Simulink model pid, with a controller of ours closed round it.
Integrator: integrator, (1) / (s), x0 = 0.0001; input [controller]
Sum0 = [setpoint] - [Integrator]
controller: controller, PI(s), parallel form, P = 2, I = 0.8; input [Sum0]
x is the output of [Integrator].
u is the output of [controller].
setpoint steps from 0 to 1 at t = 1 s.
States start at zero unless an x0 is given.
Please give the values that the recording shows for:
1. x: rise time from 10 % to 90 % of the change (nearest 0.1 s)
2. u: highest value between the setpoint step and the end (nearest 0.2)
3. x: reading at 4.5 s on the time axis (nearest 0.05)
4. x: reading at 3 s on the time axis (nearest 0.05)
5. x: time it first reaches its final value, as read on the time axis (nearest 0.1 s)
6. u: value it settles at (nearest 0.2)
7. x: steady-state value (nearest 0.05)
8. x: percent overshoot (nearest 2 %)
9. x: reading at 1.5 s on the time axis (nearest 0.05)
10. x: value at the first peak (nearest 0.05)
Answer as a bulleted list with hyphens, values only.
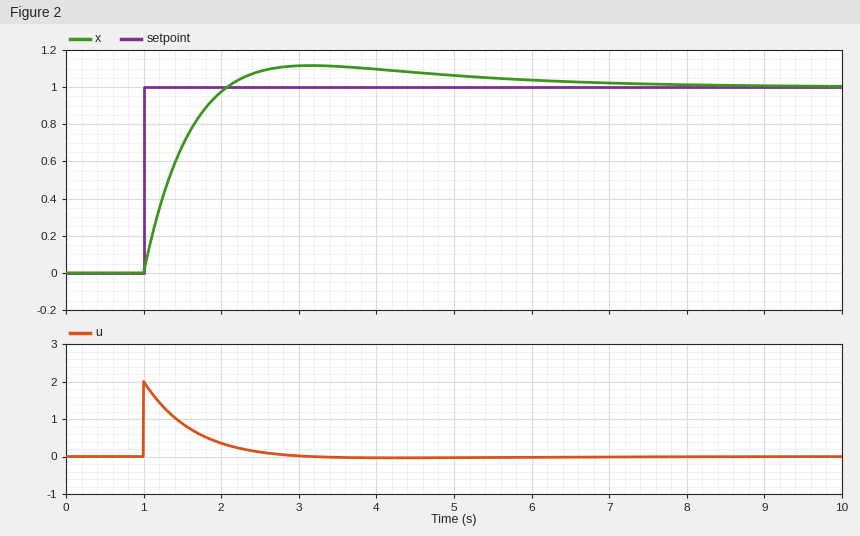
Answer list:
- 0.8 s
- 2.0
- 1.10
- 1.10
- 2.1 s
- 0.0
- 1.00
- 12 %
- 0.70
- 1.10
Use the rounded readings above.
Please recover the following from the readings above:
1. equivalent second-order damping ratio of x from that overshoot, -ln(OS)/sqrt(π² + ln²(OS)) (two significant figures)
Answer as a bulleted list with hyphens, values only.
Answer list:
- 0.56
